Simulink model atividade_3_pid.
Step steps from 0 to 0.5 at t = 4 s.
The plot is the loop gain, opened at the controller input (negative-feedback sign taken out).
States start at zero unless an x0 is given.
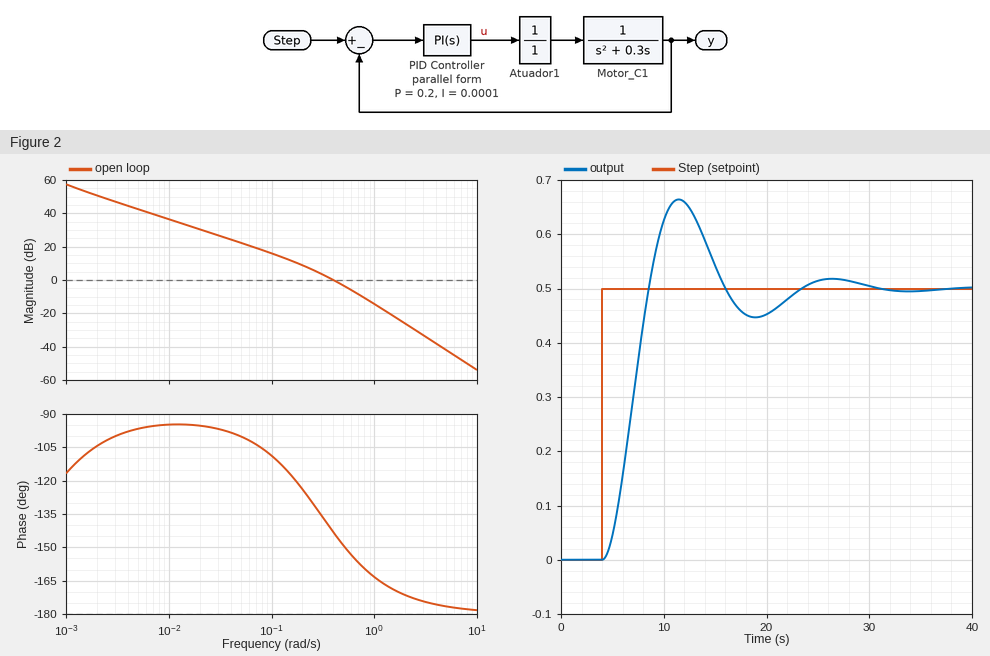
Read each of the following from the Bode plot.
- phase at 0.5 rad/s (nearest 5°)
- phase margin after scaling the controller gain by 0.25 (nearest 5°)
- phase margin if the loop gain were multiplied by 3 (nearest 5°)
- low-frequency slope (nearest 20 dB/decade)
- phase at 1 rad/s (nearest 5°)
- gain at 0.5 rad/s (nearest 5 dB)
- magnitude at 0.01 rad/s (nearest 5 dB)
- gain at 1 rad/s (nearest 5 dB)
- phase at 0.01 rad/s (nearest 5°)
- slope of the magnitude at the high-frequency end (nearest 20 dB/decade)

-150°
65°
20°
-20 dB/decade
-165°
-5 dB
35 dB
-15 dB
-95°
-40 dB/decade
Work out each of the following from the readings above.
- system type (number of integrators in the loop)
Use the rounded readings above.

1
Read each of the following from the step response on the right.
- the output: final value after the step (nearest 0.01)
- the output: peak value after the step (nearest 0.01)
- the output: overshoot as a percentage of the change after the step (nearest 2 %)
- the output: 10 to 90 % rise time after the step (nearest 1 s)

0.50
0.66
32 %
3 s
